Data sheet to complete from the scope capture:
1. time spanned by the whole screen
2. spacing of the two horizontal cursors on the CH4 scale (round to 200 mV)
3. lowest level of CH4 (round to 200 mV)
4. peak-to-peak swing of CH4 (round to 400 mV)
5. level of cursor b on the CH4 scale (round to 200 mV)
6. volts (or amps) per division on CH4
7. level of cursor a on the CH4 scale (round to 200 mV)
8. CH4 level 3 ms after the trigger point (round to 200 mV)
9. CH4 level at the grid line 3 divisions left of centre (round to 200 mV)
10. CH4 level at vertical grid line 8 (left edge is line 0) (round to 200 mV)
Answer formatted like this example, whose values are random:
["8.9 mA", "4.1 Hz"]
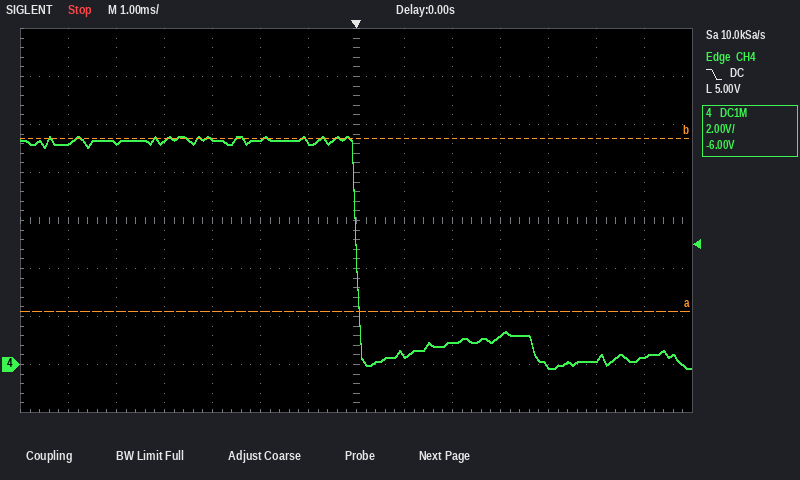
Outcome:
["14 ms", "7.2 V", "-200 mV", "9.6 V", "9.4 V", "2 V", "2.2 V", "1.2 V", "9.4 V", "400 mV"]
